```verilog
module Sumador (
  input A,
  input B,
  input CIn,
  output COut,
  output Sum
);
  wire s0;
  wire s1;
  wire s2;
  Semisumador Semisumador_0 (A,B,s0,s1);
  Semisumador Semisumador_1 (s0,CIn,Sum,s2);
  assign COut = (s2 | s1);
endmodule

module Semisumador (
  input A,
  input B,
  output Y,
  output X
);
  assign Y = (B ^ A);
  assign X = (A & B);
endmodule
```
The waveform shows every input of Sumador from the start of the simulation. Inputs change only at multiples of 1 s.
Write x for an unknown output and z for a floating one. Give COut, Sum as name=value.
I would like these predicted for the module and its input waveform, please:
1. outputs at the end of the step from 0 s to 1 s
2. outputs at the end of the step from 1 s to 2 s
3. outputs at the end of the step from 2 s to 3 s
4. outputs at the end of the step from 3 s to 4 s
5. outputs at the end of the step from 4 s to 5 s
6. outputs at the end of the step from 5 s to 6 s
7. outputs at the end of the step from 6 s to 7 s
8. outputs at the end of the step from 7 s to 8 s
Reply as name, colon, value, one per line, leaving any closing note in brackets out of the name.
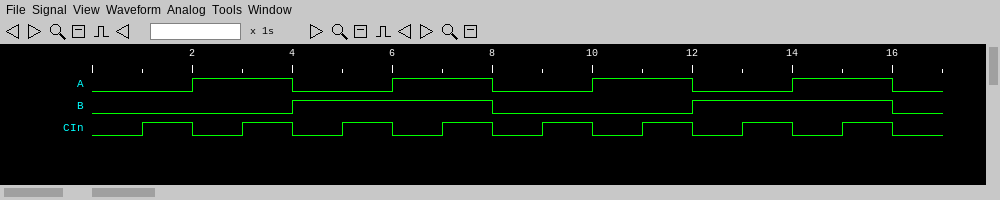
outputs at the end of the step from 0 s to 1 s: COut=0, Sum=0
outputs at the end of the step from 1 s to 2 s: COut=0, Sum=1
outputs at the end of the step from 2 s to 3 s: COut=0, Sum=1
outputs at the end of the step from 3 s to 4 s: COut=1, Sum=0
outputs at the end of the step from 4 s to 5 s: COut=0, Sum=1
outputs at the end of the step from 5 s to 6 s: COut=1, Sum=0
outputs at the end of the step from 6 s to 7 s: COut=1, Sum=0
outputs at the end of the step from 7 s to 8 s: COut=1, Sum=1
